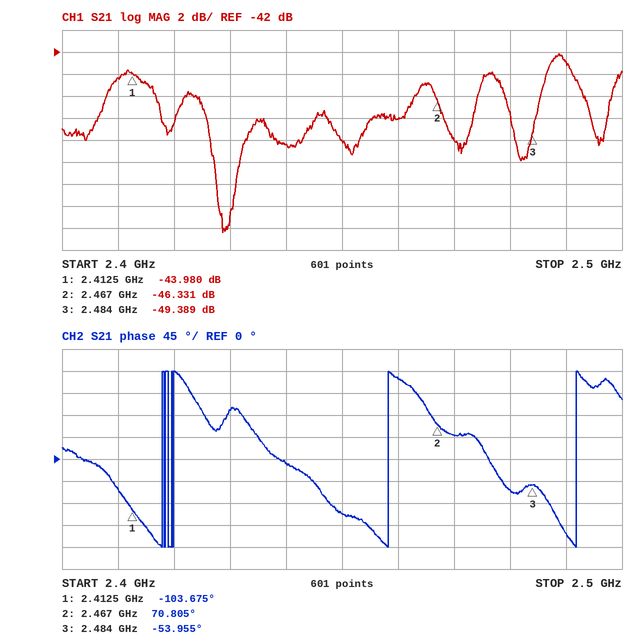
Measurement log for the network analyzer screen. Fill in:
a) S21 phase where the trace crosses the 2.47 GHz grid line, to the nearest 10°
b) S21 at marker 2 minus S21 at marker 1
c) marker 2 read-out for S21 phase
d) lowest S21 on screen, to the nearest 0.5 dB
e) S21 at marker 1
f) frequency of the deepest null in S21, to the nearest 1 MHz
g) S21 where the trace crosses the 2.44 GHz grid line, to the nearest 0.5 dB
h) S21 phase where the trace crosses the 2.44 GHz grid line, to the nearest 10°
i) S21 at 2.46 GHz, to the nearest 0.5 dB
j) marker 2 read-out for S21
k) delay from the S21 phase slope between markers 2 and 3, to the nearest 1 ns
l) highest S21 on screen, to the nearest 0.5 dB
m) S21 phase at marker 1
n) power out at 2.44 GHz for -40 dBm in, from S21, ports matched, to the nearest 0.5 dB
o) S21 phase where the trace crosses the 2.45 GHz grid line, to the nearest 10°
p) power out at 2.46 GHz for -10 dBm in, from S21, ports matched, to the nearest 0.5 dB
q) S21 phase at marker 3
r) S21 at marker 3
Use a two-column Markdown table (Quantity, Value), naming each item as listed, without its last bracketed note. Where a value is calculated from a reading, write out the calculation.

| Quantity | Value |
|---|---|
| S21 phase where the trace crosses the 2.47 GHz grid line, to the nearest 10° | 50° |
| S21 at marker 2 minus S21 at marker 1 | -46.331 − (-43.98) = -2.351 dB |
| marker 2 read-out for S21 phase | 70.805° |
| lowest S21 on screen, to the nearest 0.5 dB | -58.5 dB |
| S21 at marker 1 | -43.980 dB |
| frequency of the deepest null in S21, to the nearest 1 MHz | 2.429 GHz |
| S21 where the trace crosses the 2.44 GHz grid line, to the nearest 0.5 dB | -50.5 dB |
| S21 phase where the trace crosses the 2.44 GHz grid line, to the nearest 10° | -10° |
| S21 at 2.46 GHz, to the nearest 0.5 dB | -48.0 dB |
| marker 2 read-out for S21 | -46.331 dB |
| delay from the S21 phase slope between markers 2 and 3, to the nearest 1 ns | −(-53.955° − (70.805°))/(360° × 17 MHz) ≈ 20 ns |
| highest S21 on screen, to the nearest 0.5 dB | -42.0 dB |
| S21 phase at marker 1 | -103.675° |
| power out at 2.44 GHz for -40 dBm in, from S21, ports matched, to the nearest 0.5 dB | -40 dBm + (-50.5 dB) = -90.5 dBm |
| S21 phase where the trace crosses the 2.45 GHz grid line, to the nearest 10° | -110° |
| power out at 2.46 GHz for -10 dBm in, from S21, ports matched, to the nearest 0.5 dB | -10 dBm + (-48.0 dB) = -58.0 dBm |
| S21 phase at marker 3 | -53.955° |
| S21 at marker 3 | -49.389 dB |
